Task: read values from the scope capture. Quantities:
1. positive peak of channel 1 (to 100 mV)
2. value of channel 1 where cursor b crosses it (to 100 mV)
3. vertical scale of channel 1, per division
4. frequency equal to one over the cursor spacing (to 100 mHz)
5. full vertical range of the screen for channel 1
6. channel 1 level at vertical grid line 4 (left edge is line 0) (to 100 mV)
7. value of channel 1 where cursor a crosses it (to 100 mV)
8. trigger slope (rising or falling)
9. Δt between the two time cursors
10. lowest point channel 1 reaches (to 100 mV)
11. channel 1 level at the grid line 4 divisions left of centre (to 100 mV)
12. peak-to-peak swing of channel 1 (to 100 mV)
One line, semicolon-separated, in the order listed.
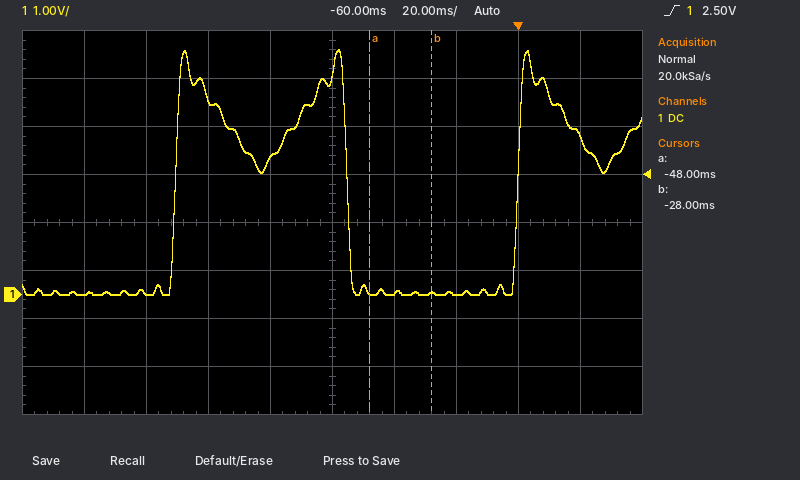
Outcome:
5.1 V; 0.0 V; 1 V; 50.0 Hz; 8 V; 2.8 V; 100 mV; rising; 20 ms; 0.0 V; 0.0 V; 5.1 V
